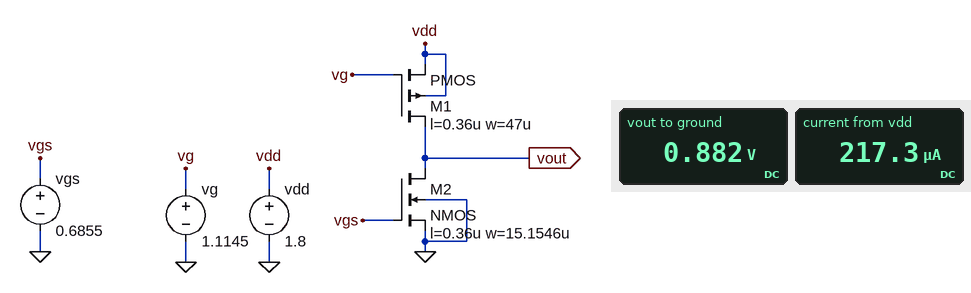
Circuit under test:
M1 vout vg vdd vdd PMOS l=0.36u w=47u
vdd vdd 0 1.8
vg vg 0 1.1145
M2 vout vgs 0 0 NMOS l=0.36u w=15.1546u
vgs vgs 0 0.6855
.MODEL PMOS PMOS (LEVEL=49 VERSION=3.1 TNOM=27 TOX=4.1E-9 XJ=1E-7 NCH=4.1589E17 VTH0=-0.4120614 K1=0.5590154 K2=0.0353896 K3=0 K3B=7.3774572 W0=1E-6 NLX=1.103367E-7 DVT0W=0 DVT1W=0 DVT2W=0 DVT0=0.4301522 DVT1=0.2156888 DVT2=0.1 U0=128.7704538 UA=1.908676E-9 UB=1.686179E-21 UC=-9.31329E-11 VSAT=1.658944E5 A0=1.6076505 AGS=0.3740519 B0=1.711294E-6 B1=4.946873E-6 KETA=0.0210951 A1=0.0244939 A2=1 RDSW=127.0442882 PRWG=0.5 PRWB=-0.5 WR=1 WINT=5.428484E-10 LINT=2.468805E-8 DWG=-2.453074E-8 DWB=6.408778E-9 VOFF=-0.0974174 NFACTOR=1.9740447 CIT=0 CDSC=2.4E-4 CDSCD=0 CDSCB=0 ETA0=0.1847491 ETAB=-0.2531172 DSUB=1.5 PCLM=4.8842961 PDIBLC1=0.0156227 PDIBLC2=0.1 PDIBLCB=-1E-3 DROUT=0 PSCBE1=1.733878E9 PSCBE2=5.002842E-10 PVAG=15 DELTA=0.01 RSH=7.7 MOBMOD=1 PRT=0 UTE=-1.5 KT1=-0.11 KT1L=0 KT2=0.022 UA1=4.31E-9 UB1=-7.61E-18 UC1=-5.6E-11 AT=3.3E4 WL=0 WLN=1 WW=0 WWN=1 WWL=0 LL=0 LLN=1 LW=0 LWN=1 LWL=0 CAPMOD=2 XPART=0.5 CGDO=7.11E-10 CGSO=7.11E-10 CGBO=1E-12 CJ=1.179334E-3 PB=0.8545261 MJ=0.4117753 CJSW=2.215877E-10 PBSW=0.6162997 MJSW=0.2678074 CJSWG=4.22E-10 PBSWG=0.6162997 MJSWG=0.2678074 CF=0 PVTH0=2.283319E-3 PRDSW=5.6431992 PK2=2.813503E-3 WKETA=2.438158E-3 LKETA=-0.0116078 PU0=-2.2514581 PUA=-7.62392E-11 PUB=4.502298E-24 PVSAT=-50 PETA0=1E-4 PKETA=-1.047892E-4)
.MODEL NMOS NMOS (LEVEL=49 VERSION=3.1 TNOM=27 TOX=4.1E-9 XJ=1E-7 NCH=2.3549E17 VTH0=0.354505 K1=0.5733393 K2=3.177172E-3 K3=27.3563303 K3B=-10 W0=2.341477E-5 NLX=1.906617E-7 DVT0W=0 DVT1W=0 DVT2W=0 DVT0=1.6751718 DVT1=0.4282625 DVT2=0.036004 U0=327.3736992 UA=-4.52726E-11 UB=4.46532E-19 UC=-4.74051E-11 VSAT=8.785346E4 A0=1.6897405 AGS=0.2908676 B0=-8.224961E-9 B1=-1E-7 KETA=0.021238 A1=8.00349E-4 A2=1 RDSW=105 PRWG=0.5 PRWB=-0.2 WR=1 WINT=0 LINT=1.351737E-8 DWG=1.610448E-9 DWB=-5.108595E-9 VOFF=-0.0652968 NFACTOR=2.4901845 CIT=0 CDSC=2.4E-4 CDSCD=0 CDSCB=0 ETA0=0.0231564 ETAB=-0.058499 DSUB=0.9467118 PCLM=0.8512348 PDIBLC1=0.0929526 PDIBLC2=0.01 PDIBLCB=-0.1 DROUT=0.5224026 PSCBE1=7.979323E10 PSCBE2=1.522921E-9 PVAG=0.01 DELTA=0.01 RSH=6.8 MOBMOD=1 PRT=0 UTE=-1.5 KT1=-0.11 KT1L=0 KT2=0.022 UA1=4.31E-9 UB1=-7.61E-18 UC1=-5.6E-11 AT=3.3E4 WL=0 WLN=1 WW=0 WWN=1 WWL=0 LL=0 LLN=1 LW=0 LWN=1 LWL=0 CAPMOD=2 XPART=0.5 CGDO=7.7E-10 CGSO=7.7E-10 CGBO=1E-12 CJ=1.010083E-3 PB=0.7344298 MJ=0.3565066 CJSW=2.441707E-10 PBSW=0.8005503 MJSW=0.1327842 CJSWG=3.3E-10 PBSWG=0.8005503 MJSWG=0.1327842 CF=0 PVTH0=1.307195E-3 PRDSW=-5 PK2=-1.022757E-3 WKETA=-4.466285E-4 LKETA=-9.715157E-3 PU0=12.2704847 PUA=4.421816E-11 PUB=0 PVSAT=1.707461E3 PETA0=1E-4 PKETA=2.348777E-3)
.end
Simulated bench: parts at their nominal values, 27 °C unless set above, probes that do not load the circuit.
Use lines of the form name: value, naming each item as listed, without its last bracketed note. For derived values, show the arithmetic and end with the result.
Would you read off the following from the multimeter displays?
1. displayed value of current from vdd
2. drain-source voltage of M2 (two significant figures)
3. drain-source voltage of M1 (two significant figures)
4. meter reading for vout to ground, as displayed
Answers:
displayed value of current from vdd: 217.3 µA
drain-source voltage of M2: 882 mV = 880 mV
drain-source voltage of M1: 882 mV - 1.8 V = -920 mV
meter reading for vout to ground, as displayed: 0.882 V
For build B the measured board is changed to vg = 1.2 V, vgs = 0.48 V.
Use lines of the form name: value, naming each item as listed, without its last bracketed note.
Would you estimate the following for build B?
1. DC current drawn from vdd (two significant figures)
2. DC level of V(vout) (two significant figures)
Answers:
DC current drawn from vdd: 8.1 µA
DC level of V(vout): 1.8 V
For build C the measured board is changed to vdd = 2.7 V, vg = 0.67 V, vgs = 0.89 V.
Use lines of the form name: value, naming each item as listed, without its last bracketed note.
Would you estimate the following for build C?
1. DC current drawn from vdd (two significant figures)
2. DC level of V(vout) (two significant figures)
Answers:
DC current drawn from vdd: 860 µA
DC level of V(vout): 2.6 V
